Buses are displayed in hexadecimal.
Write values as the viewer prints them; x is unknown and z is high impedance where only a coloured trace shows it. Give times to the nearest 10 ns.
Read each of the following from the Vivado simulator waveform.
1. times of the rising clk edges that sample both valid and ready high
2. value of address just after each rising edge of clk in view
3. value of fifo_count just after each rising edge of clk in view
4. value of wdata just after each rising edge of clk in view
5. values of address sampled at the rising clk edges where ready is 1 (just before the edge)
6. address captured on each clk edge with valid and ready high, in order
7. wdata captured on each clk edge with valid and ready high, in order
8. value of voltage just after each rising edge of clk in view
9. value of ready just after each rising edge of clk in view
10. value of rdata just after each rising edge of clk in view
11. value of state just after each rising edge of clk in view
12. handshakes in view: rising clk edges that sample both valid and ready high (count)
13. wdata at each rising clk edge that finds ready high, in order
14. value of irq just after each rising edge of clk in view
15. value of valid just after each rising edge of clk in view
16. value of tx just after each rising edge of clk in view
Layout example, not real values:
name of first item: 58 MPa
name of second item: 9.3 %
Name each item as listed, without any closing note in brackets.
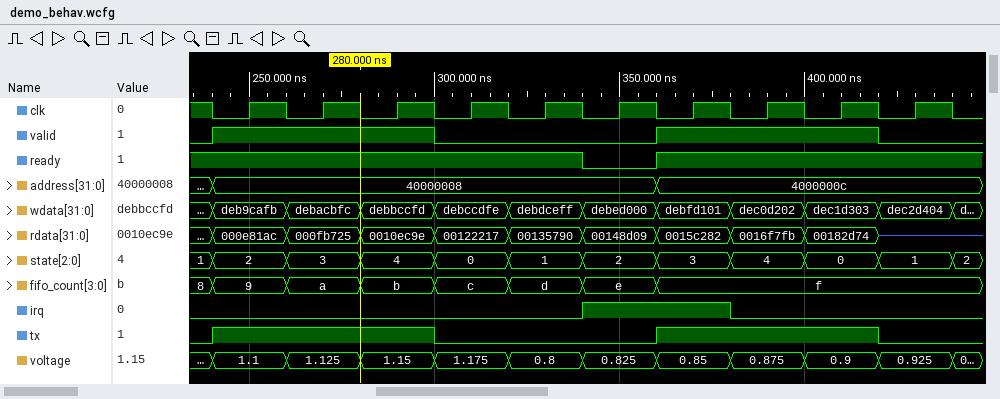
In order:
times of the rising clk edges that sample both valid and ready high: 250 ns, 270 ns, 290 ns, 370 ns, 390 ns, 410 ns
value of address just after each rising edge of clk in view: 40000008, 40000008, 40000008, 40000008, 40000008, 40000008, 4000000c, 4000000c, 4000000c, 4000000c
value of fifo_count just after each rising edge of clk in view: 9, a, b, c, d, e, f, f, f, f
value of wdata just after each rising edge of clk in view: deb9cafb, debacbfc, debbccfd, debccdfe, debdceff, debed000, debfd101, dec0d202, dec1d303, dec2d404
values of address sampled at the rising clk edges where ready is 1: 40000008, 40000008, 40000008, 40000008, 40000008, 4000000c, 4000000c, 4000000c, 4000000c
address captured on each clk edge with valid and ready high, in order: 40000008, 40000008, 40000008, 4000000c, 4000000c, 4000000c
wdata captured on each clk edge with valid and ready high, in order: deb9cafb, debacbfc, debbccfd, debfd101, dec0d202, dec1d303
value of voltage just after each rising edge of clk in view: 1.1, 1.125, 1.15, 1.175, 0.8, 0.825, 0.85, 0.875, 0.9, 0.925
value of ready just after each rising edge of clk in view: 1 1 1 1 1 0 1 1 1 1
value of rdata just after each rising edge of clk in view: 000e81ac, 000fb725, 0010ec9e, 00122217, 00135790, 00148d09, 0015c282, 0016f7fb, 00182d74, z
value of state just after each rising edge of clk in view: 2, 3, 4, 0, 1, 2, 3, 4, 0, 1
handshakes in view: rising clk edges that sample both valid and ready high: 6
wdata at each rising clk edge that finds ready high, in order: deb9cafb, debacbfc, debbccfd, debccdfe, debdceff, debfd101, dec0d202, dec1d303, dec2d404
value of irq just after each rising edge of clk in view: 0 0 0 0 0 1 1 0 0 0
value of valid just after each rising edge of clk in view: 1 1 1 0 0 0 1 1 1 0
value of tx just after each rising edge of clk in view: 1 1 1 0 0 0 1 1 1 0
